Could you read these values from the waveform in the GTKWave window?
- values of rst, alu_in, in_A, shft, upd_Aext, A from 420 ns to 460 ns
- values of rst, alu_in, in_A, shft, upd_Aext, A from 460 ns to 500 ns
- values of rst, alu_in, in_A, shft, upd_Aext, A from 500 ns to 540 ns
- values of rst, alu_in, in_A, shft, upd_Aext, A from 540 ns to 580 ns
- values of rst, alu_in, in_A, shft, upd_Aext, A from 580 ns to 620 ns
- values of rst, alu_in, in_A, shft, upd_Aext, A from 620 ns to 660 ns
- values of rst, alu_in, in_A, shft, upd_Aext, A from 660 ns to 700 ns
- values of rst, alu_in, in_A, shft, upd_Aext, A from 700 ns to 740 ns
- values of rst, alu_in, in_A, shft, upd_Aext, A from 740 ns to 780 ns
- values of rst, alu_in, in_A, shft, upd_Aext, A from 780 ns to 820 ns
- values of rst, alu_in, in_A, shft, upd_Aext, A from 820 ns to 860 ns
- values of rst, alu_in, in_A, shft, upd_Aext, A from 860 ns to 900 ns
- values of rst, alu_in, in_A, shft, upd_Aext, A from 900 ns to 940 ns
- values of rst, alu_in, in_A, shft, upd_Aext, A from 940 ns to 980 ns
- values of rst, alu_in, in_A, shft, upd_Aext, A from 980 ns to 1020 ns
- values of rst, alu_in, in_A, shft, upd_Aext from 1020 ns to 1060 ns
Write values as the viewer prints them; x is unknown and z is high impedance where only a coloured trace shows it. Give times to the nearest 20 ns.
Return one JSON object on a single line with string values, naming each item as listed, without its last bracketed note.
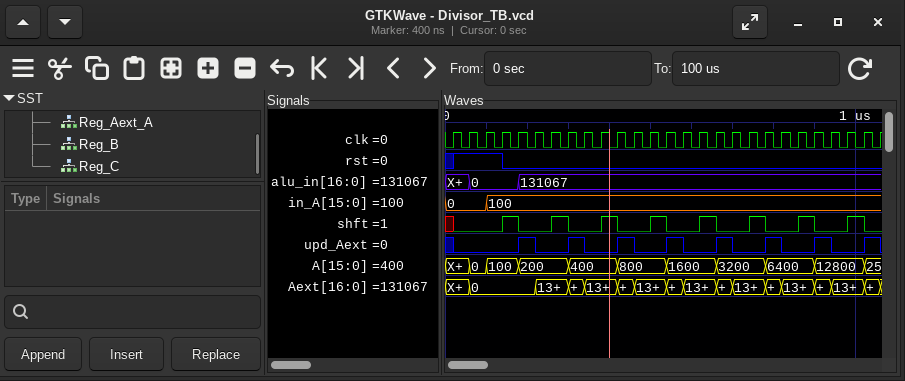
{"values of rst, alu_in, in_A, shft, upd_Aext, A from 420 ns to 460 ns": "rst=0, alu_in=131067, in_A=100, shft=0, upd_Aext=1, A=800", "values of rst, alu_in, in_A, shft, upd_Aext, A from 460 ns to 500 ns": "rst=0, alu_in=131067, in_A=100, shft=0, upd_Aext=0, A=800", "values of rst, alu_in, in_A, shft, upd_Aext, A from 500 ns to 540 ns": "rst=0, alu_in=131067, in_A=100, shft=1, upd_Aext=0, A=800", "values of rst, alu_in, in_A, shft, upd_Aext, A from 540 ns to 580 ns": "rst=0, alu_in=131067, in_A=100, shft=0, upd_Aext=1, A=1600", "values of rst, alu_in, in_A, shft, upd_Aext, A from 580 ns to 620 ns": "rst=0, alu_in=131067, in_A=100, shft=0, upd_Aext=0, A=1600", "values of rst, alu_in, in_A, shft, upd_Aext, A from 620 ns to 660 ns": "rst=0, alu_in=131067, in_A=100, shft=1, upd_Aext=0, A=1600", "values of rst, alu_in, in_A, shft, upd_Aext, A from 660 ns to 700 ns": "rst=0, alu_in=131067, in_A=100, shft=0, upd_Aext=1, A=3200", "values of rst, alu_in, in_A, shft, upd_Aext, A from 700 ns to 740 ns": "rst=0, alu_in=131067, in_A=100, shft=0, upd_Aext=0, A=3200", "values of rst, alu_in, in_A, shft, upd_Aext, A from 740 ns to 780 ns": "rst=0, alu_in=131067, in_A=100, shft=1, upd_Aext=0, A=3200", "values of rst, alu_in, in_A, shft, upd_Aext, A from 780 ns to 820 ns": "rst=0, alu_in=131067, in_A=100, shft=0, upd_Aext=1, A=6400", "values of rst, alu_in, in_A, shft, upd_Aext, A from 820 ns to 860 ns": "rst=0, alu_in=131067, in_A=100, shft=0, upd_Aext=0, A=6400", "values of rst, alu_in, in_A, shft, upd_Aext, A from 860 ns to 900 ns": "rst=0, alu_in=131067, in_A=100, shft=1, upd_Aext=0, A=6400", "values of rst, alu_in, in_A, shft, upd_Aext, A from 900 ns to 940 ns": "rst=0, alu_in=131067, in_A=100, shft=0, upd_Aext=1, A=12800", "values of rst, alu_in, in_A, shft, upd_Aext, A from 940 ns to 980 ns": "rst=0, alu_in=131067, in_A=100, shft=0, upd_Aext=0, A=12800", "values of rst, alu_in, in_A, shft, upd_Aext, A from 980 ns to 1020 ns": "rst=0, alu_in=131067, in_A=100, shft=1, upd_Aext=0, A=12800", "values of rst, alu_in, in_A, shft, upd_Aext from 1020 ns to 1060 ns": "rst=0, alu_in=131067, in_A=100, shft=0, upd_Aext=1"}
